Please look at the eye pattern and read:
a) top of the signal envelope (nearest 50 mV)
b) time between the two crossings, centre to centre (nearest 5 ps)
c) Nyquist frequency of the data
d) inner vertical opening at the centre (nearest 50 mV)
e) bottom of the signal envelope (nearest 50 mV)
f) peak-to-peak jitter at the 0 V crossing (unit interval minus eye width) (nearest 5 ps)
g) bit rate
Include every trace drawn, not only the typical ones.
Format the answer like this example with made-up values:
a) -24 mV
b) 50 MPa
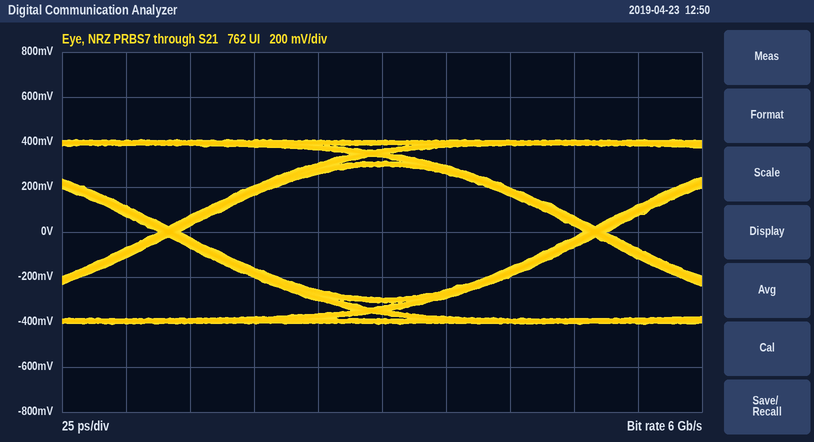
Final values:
a) 400 mV
b) 165 ps
c) 3 GHz
d) 600 mV
e) -400 mV
f) 10 ps
g) 6 Gb/s
